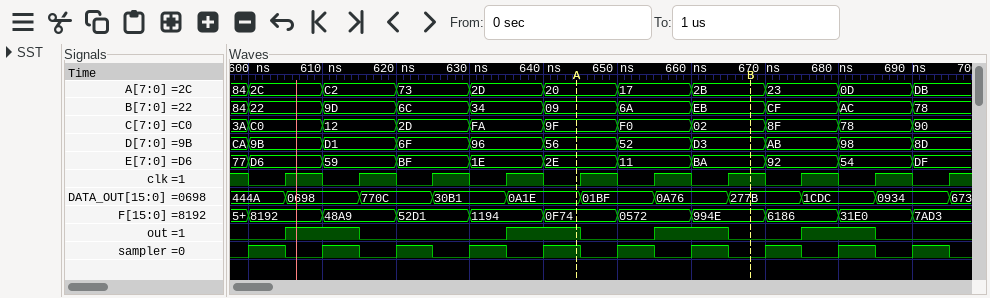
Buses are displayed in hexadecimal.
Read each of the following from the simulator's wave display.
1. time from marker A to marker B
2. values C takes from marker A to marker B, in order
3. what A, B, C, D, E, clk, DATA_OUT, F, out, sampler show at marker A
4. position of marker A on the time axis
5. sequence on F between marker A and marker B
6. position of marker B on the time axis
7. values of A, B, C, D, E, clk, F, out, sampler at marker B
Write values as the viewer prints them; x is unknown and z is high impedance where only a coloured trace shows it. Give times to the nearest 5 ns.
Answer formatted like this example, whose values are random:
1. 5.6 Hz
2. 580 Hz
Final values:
1. 25 ns
2. 9F, F0, 02
3. A=20, B=09, C=9F, D=56, E=2E, clk=0, DATA_OUT=0A1E, F=0F74, out=1, sampler=1
4. 645 ns
5. 0F74, 0572, 994E
6. 670 ns
7. A=2B, B=EB, C=02, D=D3, E=BA, clk=1, F=994E, out=0, sampler=0
